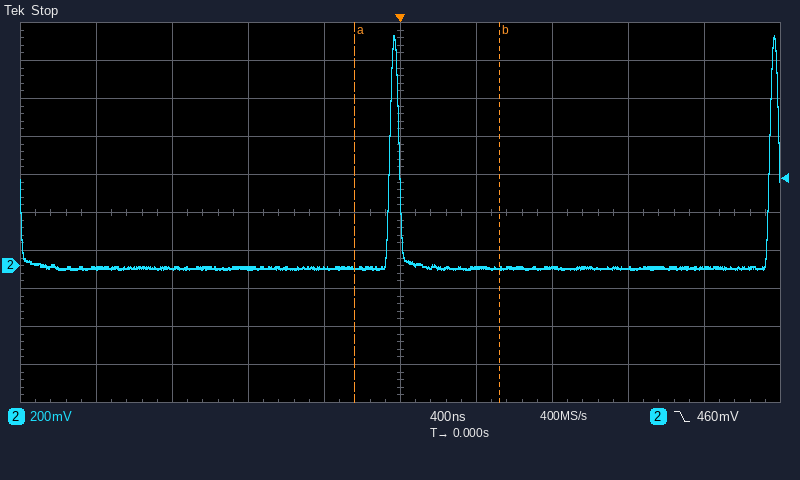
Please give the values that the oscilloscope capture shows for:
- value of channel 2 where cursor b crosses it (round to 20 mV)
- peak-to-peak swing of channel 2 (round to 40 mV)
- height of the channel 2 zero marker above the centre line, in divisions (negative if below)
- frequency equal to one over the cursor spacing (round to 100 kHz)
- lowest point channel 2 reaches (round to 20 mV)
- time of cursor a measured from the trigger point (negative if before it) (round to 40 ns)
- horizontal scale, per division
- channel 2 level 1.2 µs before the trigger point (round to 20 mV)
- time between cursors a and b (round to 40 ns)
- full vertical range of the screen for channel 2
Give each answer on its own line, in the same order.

-20 mV
1.24 V
-1.4 div
1.3 MHz
-20 mV
-240 ns
400 ns
-20 mV
760 ns
2 V
